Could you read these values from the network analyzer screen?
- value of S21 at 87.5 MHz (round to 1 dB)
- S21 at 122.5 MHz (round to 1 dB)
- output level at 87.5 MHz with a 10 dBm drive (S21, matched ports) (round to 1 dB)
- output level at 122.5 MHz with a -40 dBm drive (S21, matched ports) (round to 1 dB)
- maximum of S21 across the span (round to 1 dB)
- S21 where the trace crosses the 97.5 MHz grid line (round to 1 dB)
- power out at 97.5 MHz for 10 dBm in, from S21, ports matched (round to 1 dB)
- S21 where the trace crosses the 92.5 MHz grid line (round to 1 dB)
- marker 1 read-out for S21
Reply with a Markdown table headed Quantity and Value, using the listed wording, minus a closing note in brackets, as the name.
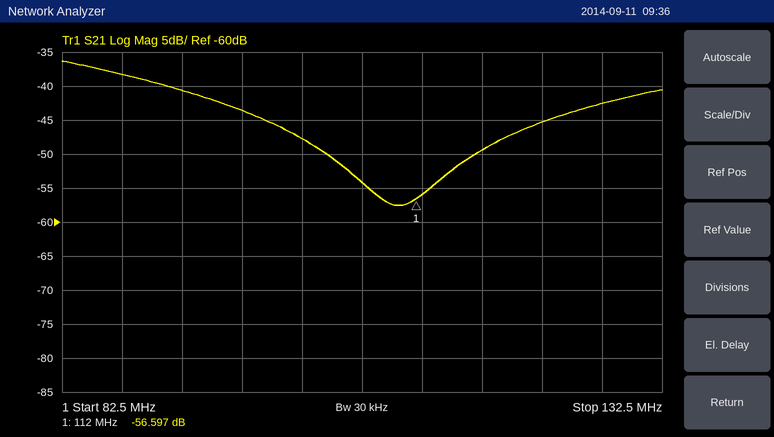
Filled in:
| Quantity | Value |
|---|---|
| value of S21 at 87.5 MHz | -38 dB |
| S21 at 122.5 MHz | -45 dB |
| output level at 87.5 MHz with a 10 dBm drive (S21, matched ports) | -28 dBm |
| output level at 122.5 MHz with a -40 dBm drive (S21, matched ports) | -85 dBm |
| maximum of S21 across the span | -36 dB |
| S21 where the trace crosses the 97.5 MHz grid line | -44 dB |
| power out at 97.5 MHz for 10 dBm in, from S21, ports matched | -34 dBm |
| S21 where the trace crosses the 92.5 MHz grid line | -41 dB |
| marker 1 read-out for S21 | -56.597 dB |
